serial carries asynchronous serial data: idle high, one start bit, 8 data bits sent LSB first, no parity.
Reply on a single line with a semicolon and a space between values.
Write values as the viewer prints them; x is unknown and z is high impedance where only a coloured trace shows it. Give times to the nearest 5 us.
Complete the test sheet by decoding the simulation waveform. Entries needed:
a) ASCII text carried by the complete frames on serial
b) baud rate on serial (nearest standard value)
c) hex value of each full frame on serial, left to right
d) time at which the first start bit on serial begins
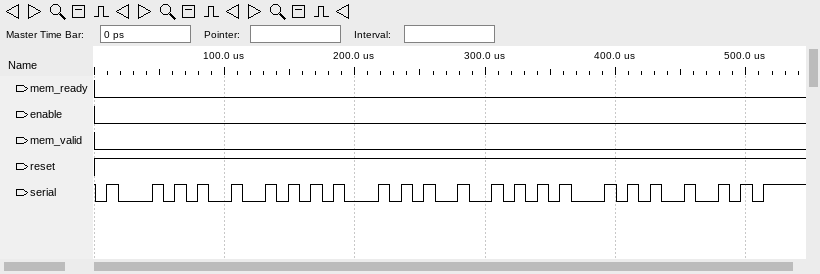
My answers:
"QRQRQR"; 115200 baud; 51, 52, 51, 52, 51, 52; 0 us
